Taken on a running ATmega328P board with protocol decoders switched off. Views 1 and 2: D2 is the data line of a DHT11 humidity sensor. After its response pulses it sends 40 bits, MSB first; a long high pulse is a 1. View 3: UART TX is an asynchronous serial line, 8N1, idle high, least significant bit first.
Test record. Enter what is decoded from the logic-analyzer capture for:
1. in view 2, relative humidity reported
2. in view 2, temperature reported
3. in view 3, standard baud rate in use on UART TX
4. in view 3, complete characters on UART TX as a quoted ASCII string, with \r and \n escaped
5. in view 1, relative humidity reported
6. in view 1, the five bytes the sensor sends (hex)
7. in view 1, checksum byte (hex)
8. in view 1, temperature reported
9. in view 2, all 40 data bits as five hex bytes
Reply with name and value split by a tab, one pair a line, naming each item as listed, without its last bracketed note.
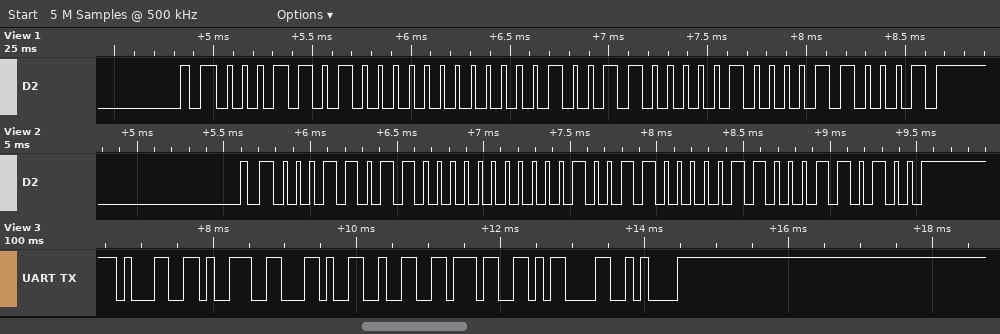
in view 2, relative humidity reported	27 %
in view 2, temperature reported	19.6 °C
in view 3, standard baud rate in use on UART TX	9600 baud
in view 3, complete characters on UART TX as a quoted ASCII string, with \r and \n escaped	"19,27\r\n"
in view 1, relative humidity reported	26 %
in view 1, the five bytes the sensor sends	1A 00 13 04 31
in view 1, checksum byte	0x31
in view 1, temperature reported	19.4 °C
in view 2, all 40 data bits as five hex bytes	1B 00 13 06 34
